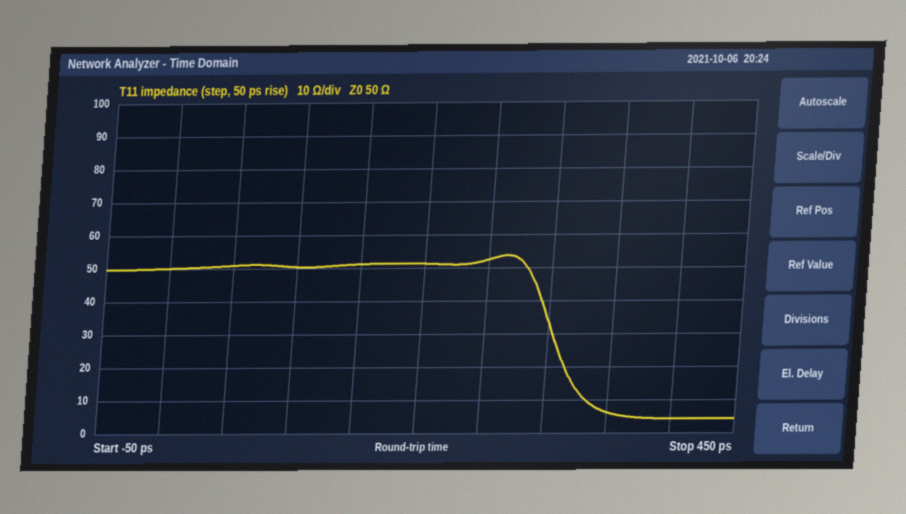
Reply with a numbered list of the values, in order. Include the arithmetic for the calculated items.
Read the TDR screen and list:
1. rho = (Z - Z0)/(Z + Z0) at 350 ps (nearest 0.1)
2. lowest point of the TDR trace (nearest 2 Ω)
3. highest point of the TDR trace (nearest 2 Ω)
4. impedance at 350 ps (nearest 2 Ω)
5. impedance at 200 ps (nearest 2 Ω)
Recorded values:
1. (6 − 50)/(6 + 50) ≈ -0.8
2. 4 Ω
3. 54 Ω
4. 6 Ω
5. 52 Ω
